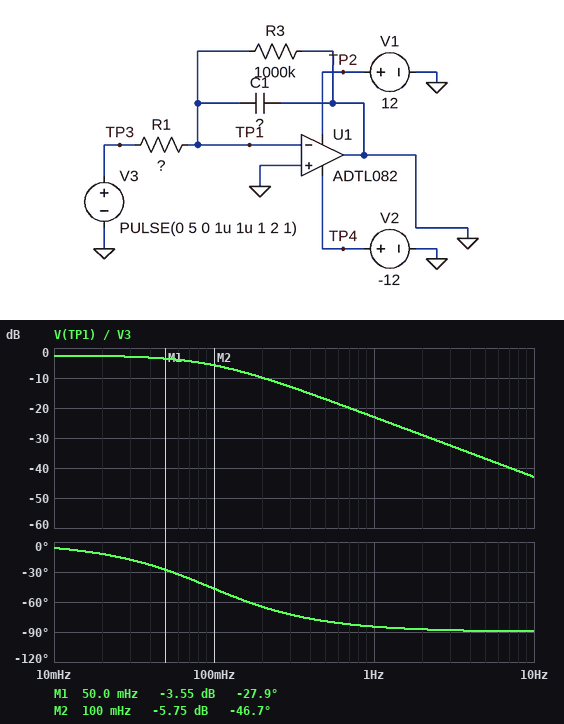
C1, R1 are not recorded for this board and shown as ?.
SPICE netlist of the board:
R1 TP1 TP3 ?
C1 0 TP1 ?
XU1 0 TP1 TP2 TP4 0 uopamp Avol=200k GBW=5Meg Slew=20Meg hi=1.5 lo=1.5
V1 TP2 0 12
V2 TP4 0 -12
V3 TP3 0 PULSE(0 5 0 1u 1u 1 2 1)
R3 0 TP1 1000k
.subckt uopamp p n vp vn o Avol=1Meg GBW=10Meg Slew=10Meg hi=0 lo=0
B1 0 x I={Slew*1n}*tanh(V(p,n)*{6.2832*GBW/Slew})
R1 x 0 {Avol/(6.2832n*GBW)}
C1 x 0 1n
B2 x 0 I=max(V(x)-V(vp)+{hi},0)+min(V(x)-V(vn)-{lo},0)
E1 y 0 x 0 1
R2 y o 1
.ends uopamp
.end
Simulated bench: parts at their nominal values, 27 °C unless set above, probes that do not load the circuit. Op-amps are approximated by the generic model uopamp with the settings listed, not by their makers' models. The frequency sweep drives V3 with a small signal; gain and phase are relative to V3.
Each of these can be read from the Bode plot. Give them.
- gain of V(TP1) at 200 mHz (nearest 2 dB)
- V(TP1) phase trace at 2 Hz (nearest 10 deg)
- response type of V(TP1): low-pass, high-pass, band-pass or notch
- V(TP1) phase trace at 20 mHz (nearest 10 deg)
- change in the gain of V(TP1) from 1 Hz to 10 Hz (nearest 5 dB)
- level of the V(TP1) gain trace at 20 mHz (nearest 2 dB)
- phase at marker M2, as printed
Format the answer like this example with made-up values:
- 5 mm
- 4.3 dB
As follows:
- -10 dB
- -90 deg
- low-pass
- -10 deg
- -20 dB
- -2 dB
- -46.7 deg
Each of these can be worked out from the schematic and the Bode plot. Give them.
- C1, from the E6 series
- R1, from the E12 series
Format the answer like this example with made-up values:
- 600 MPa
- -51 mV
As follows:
- 6.8 µF
- 330 kΩ
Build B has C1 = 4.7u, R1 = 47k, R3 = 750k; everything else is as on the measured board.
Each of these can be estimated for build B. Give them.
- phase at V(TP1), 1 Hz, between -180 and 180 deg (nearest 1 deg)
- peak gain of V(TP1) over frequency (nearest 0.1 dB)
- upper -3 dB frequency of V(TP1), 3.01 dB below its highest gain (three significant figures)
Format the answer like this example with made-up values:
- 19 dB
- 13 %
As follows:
- -53 deg
- -0.5 dB
- 766 mHz
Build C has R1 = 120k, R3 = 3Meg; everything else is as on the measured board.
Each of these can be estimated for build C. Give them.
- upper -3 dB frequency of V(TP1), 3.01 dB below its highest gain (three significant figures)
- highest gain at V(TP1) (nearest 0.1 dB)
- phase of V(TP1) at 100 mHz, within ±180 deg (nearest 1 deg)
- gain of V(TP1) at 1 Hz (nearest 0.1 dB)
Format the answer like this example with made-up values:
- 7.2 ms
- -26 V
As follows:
- 203 mHz
- -0.3 dB
- -26 deg
- -14.4 dB
